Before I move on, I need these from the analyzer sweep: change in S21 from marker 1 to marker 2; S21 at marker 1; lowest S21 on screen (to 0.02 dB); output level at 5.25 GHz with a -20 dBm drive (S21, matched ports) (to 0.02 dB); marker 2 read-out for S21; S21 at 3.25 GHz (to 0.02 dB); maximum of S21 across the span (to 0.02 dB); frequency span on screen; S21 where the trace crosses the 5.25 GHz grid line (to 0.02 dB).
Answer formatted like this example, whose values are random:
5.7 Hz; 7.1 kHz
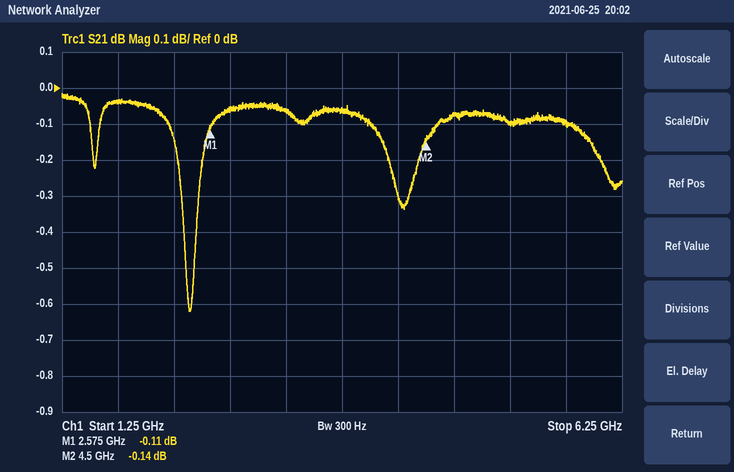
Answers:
-0.03 dB; -0.11 dB; -0.62 dB; -20.10 dBm; -0.14 dB; -0.06 dB; -0.02 dB; 5 GHz; -0.10 dB
